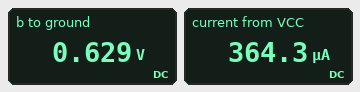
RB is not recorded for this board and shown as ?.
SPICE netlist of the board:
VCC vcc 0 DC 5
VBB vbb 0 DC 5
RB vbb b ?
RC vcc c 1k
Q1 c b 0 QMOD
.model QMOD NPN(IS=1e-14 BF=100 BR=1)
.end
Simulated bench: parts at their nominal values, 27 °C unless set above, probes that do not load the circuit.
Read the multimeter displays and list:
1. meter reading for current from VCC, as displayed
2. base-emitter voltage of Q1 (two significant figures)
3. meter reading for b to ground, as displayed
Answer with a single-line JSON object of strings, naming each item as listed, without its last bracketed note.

{"meter reading for current from VCC, as displayed": "364.3 µA", "base-emitter voltage of Q1": "630 mV", "meter reading for b to ground, as displayed": "0.629 V"}
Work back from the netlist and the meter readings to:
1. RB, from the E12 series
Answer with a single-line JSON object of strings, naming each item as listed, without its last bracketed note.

{"RB, from the E12 series": "1.2 MΩ"}
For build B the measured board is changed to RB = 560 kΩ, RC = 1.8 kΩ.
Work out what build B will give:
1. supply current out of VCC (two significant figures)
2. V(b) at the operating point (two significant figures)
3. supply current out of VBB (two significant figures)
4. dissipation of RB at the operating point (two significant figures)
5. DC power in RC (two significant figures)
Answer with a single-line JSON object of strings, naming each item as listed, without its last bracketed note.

{"supply current out of VCC": "780 µA", "V(b) at the operating point": "650 mV", "supply current out of VBB": "7.8 µA", "dissipation of RB at the operating point": "34 µW", "DC power in RC": "1.1 mW"}
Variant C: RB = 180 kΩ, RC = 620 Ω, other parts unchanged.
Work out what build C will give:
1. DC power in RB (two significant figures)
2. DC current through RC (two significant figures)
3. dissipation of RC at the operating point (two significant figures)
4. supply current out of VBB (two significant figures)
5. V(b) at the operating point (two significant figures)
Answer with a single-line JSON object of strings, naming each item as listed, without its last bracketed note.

{"DC power in RB": "100 µW", "DC current through RC": "2.4 mA", "dissipation of RC at the operating point": "3.6 mW", "supply current out of VBB": "24 µA", "V(b) at the operating point": "680 mV"}
